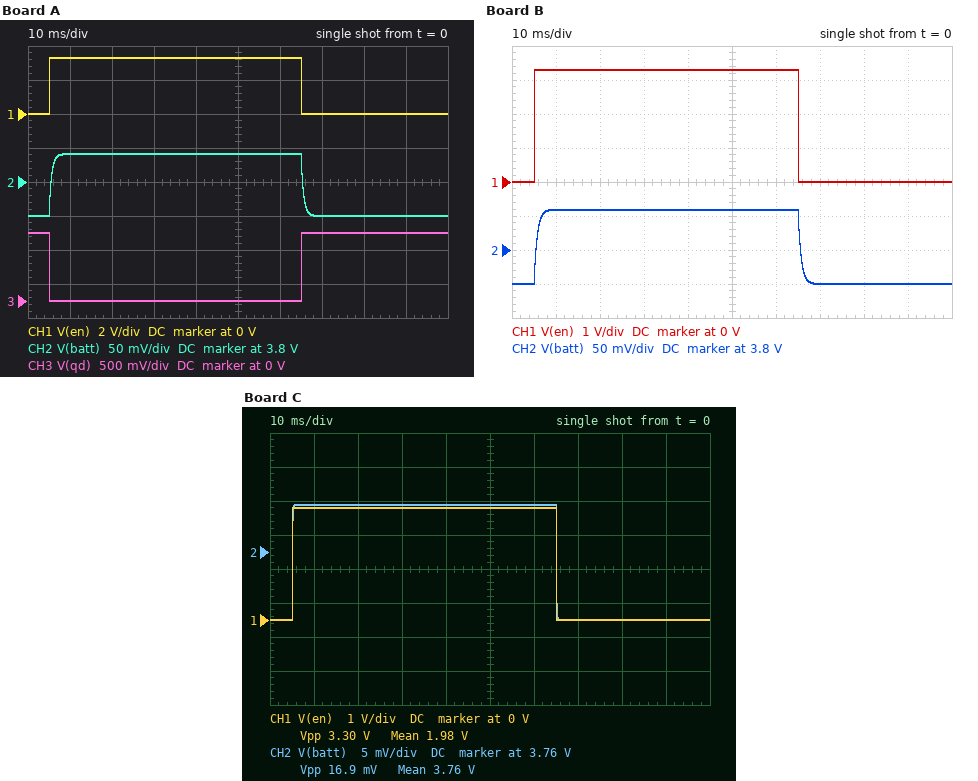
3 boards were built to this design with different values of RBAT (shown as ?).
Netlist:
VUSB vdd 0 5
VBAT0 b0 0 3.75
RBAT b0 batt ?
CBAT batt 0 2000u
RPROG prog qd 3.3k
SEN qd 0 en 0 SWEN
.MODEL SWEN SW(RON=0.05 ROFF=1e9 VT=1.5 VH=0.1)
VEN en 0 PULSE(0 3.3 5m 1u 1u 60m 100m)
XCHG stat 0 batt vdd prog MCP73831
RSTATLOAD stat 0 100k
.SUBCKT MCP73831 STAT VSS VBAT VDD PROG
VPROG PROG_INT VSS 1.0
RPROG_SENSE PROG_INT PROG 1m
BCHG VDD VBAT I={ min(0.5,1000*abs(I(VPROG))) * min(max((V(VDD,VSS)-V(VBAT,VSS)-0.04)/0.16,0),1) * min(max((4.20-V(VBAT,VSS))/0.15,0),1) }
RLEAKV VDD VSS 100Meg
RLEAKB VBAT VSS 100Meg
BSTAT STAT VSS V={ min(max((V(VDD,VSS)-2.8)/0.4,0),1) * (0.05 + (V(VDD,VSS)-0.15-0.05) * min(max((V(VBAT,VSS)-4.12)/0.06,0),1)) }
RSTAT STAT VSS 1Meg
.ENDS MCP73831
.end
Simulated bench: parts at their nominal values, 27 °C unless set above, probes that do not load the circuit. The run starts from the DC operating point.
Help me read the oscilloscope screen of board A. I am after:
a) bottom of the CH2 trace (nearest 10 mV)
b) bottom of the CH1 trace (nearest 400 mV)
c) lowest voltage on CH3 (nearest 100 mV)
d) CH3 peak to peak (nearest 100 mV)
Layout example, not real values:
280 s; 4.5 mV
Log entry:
3.75 V; 0 V; 0 V; 1.0 V
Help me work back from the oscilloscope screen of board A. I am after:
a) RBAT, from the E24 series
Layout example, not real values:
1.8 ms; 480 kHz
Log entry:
0.3 Ω
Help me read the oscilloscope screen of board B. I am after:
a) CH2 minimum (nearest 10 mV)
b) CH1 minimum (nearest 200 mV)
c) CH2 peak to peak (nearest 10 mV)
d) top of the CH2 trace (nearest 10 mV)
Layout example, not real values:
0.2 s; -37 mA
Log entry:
3.75 V; 0 V; 110 mV; 3.86 V
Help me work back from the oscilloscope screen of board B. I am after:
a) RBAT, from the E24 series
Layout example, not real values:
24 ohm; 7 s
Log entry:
0.36 Ω
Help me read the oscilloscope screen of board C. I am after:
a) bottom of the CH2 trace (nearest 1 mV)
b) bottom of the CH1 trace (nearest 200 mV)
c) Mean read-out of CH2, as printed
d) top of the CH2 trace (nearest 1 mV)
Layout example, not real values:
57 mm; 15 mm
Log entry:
3.750 V; 0 V; 3.76 V; 3.767 V
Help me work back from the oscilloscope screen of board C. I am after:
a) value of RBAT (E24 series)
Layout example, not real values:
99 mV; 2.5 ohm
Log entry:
0.056 Ω
